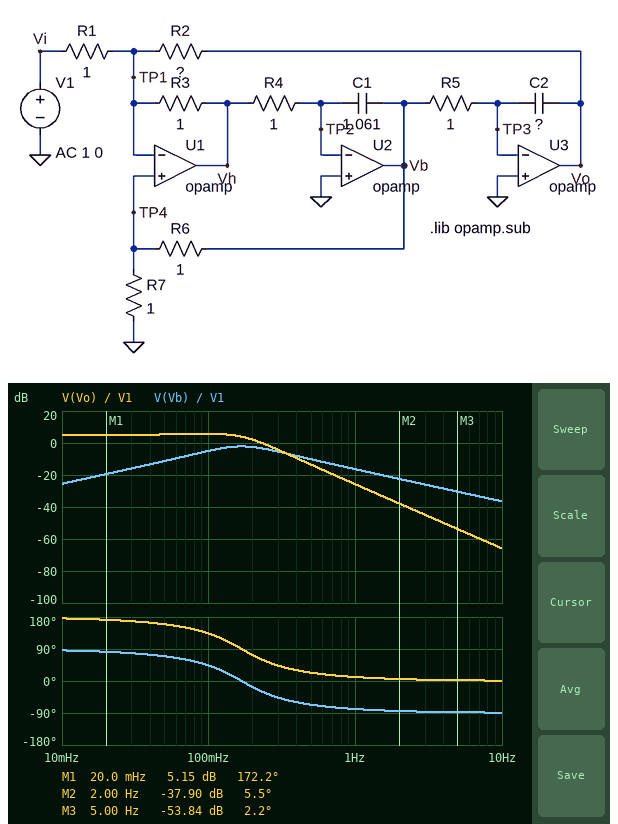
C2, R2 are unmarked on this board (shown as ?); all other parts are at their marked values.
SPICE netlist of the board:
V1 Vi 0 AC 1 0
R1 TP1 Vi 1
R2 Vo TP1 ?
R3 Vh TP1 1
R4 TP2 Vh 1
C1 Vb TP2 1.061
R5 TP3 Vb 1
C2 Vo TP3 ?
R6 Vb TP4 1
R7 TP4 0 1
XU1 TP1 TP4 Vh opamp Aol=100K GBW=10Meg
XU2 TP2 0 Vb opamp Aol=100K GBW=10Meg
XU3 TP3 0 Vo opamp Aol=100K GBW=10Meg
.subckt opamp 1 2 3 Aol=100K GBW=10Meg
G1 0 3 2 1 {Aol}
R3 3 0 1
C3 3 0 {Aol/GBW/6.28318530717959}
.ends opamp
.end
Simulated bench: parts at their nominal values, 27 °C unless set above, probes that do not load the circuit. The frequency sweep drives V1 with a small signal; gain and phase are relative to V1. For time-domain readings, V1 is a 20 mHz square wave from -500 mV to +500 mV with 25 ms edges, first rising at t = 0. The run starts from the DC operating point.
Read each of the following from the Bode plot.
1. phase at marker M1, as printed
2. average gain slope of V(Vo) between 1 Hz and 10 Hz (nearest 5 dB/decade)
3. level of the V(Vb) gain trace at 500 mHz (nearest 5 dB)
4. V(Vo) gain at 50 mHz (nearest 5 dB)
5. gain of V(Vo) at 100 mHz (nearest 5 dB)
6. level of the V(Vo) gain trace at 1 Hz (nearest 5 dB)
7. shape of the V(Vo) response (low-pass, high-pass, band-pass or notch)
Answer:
172.2 deg
-40 dB/decade
-10 dB
5 dB
5 dB
-25 dB
low-pass
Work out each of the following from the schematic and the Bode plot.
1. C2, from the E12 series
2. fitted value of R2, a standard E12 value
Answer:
470 mF
1.8 Ω
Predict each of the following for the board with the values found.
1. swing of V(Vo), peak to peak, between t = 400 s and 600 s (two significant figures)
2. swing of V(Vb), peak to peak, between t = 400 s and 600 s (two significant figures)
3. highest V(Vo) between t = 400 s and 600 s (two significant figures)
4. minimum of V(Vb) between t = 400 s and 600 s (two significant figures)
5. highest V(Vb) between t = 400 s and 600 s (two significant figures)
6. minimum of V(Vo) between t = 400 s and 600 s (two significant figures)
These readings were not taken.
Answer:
2.2 V
920 mV
1.1 V
-460 mV
460 mV
-1.1 V
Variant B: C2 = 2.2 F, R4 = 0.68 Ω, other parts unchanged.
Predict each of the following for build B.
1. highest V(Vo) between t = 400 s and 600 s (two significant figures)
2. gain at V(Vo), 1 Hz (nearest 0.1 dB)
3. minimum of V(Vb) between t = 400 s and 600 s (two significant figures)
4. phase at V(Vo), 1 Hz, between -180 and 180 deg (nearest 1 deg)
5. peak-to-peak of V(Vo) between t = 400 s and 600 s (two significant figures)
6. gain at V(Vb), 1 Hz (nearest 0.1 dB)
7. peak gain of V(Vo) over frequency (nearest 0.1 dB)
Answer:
890 mV
-36.2 dB
-640 mV
16 deg
1.8 V
-13.4 dB
5.1 dB
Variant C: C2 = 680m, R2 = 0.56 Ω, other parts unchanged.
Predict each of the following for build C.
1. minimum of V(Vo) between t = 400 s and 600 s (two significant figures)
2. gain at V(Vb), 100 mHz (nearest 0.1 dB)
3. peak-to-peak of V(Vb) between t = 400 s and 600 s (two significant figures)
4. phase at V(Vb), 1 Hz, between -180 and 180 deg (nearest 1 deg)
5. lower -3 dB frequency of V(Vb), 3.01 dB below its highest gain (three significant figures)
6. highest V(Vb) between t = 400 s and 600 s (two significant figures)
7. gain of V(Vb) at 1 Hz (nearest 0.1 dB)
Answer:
-350 mV
-12.0 dB
620 mV
-73 deg
146 mHz
310 mV
-16.3 dB
